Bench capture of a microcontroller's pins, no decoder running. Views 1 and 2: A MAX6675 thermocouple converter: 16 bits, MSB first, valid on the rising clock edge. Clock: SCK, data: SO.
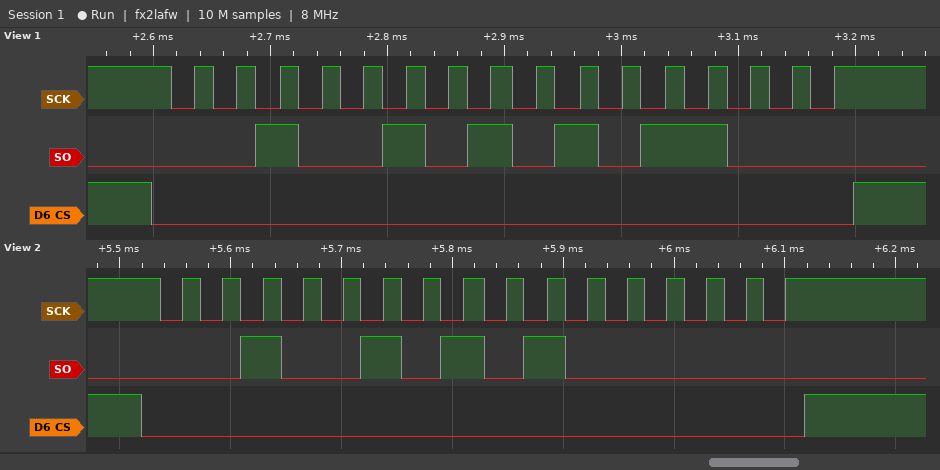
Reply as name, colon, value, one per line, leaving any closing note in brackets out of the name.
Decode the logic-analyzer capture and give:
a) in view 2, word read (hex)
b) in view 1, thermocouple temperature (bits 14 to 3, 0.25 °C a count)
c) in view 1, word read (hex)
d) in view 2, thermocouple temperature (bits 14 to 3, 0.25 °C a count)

in view 2, word read: 0x2540
in view 1, thermocouple temperature: 298.75 °C
in view 1, word read: 0x2558
in view 2, thermocouple temperature: 298.00 °C
